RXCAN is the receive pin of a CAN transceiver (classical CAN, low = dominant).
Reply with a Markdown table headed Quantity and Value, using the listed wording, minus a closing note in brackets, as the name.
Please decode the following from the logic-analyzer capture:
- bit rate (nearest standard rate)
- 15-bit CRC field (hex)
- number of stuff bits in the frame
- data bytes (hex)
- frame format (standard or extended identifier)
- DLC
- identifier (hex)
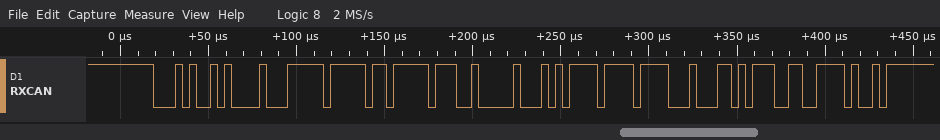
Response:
| Quantity | Value |
|---|---|
| bit rate | 250 kbit/s |
| 15-bit CRC field | 0x4CF4 |
| number of stuff bits in the frame | 4 |
| data bytes | FF F7 F9 00 AF 7B C4 6B |
| frame format | standard |
| DLC | 8 |
| identifier | 0x14A |
